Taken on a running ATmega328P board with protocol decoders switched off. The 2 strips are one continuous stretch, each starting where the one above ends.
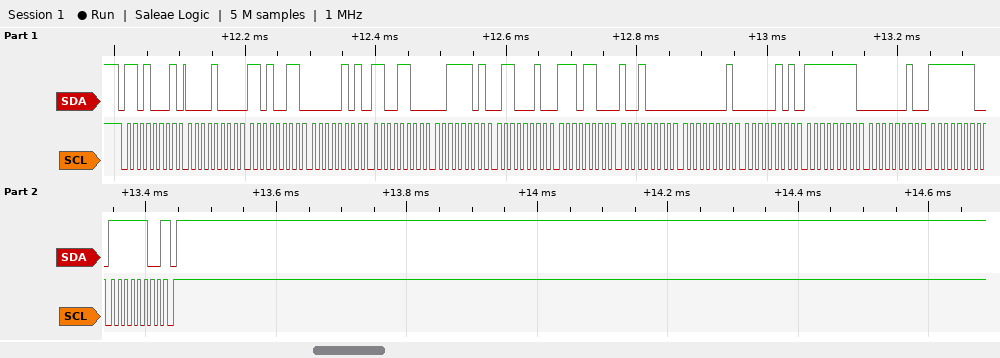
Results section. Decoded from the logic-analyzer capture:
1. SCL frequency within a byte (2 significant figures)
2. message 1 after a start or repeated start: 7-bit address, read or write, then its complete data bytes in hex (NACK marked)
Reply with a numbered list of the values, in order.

1. 100 kHz
2. 0x68 read: 08 D3 05 CC 3D 62 EC 90 01 05 FF 02 FE FC NACK
